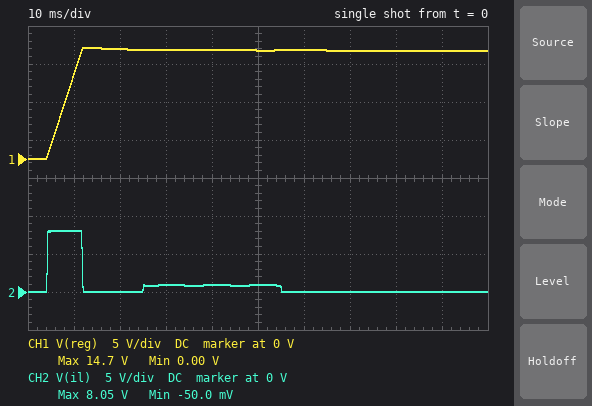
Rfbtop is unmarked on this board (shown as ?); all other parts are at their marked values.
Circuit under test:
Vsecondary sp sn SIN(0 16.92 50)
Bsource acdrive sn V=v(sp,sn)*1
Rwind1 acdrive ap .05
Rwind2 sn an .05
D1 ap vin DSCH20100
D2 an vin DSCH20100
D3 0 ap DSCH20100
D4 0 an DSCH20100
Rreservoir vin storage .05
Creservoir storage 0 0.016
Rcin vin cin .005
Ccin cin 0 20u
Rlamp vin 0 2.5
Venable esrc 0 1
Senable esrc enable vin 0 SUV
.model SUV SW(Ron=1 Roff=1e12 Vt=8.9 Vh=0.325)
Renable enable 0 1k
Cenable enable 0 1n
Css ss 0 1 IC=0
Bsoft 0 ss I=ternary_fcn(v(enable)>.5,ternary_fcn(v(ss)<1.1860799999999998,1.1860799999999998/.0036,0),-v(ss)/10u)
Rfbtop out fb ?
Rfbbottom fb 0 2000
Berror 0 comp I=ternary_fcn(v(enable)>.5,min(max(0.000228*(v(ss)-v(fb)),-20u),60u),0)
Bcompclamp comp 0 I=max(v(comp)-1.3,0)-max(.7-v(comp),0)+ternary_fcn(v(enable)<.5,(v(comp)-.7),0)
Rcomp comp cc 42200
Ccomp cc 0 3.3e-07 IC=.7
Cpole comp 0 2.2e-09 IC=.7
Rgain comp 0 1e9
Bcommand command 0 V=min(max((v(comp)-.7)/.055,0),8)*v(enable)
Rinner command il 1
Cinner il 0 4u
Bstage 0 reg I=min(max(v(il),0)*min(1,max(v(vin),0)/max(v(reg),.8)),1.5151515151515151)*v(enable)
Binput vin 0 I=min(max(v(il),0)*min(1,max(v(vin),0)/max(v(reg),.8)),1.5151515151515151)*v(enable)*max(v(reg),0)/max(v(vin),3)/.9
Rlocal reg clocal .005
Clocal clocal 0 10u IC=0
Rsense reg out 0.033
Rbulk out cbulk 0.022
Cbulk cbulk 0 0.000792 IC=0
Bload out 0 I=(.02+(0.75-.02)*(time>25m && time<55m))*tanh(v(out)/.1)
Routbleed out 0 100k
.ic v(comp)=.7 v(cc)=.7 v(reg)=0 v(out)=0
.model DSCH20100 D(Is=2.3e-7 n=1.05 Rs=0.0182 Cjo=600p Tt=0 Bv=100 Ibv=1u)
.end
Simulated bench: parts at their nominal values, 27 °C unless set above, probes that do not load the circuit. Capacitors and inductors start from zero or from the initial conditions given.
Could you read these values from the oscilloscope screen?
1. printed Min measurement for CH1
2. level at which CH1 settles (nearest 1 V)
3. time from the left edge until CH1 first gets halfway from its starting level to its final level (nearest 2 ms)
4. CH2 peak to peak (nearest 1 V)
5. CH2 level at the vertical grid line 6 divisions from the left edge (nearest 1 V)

0.00 V
14 V
8 ms
8 V
0 V
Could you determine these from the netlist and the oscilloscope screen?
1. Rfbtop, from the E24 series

22 kΩ
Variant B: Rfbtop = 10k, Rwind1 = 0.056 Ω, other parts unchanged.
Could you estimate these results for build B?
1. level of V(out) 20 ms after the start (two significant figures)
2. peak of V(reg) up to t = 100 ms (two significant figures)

7.2 V
7.4 V
